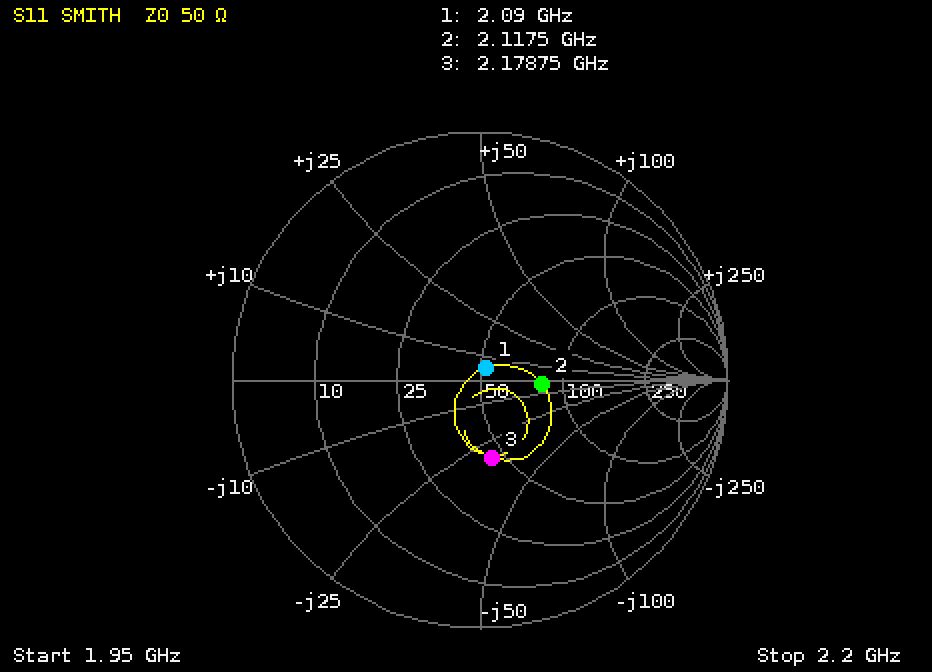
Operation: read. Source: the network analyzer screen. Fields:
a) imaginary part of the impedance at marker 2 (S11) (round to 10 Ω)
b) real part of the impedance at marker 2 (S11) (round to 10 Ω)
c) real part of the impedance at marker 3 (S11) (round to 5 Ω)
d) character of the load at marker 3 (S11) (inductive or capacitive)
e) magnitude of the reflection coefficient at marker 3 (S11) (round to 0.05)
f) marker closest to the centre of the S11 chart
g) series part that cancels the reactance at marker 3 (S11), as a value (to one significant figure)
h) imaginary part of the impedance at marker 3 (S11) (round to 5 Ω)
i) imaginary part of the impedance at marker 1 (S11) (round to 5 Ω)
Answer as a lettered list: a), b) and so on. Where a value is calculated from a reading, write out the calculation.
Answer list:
a) 0 Ω
b) 80 Ω
c) 45 Ω
d) capacitive
e) 0.30
f) marker 1
g) L = 30 Ω/(2π × 2.17875 GHz) ≈ 2 nH
h) -30 Ω
i) +5 Ω
